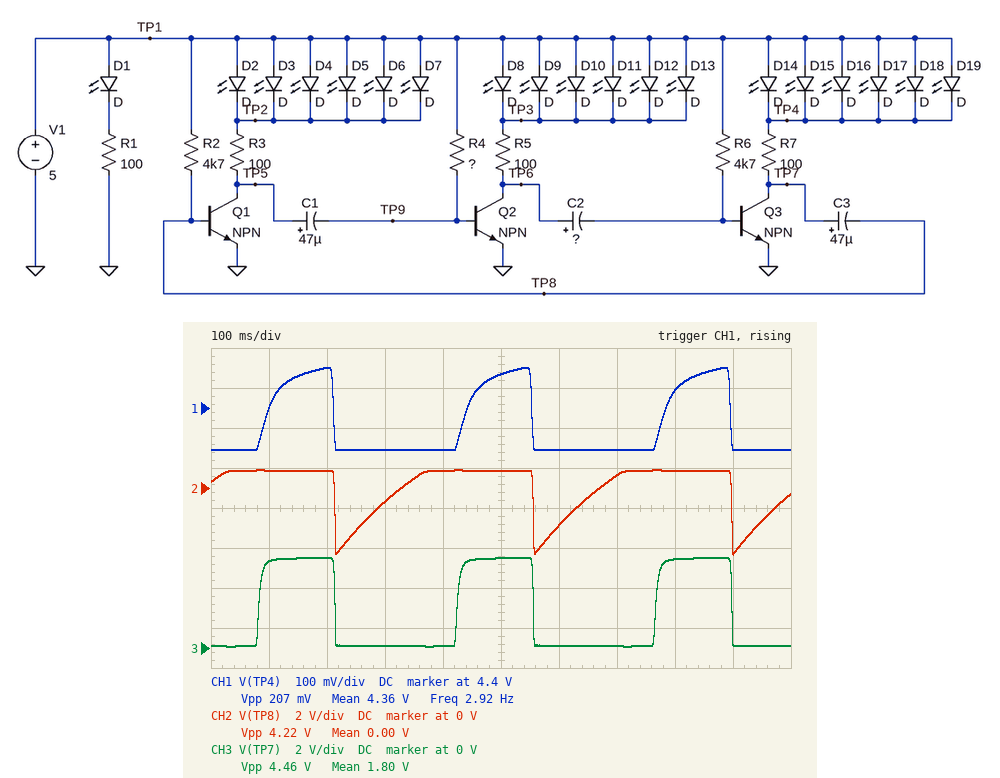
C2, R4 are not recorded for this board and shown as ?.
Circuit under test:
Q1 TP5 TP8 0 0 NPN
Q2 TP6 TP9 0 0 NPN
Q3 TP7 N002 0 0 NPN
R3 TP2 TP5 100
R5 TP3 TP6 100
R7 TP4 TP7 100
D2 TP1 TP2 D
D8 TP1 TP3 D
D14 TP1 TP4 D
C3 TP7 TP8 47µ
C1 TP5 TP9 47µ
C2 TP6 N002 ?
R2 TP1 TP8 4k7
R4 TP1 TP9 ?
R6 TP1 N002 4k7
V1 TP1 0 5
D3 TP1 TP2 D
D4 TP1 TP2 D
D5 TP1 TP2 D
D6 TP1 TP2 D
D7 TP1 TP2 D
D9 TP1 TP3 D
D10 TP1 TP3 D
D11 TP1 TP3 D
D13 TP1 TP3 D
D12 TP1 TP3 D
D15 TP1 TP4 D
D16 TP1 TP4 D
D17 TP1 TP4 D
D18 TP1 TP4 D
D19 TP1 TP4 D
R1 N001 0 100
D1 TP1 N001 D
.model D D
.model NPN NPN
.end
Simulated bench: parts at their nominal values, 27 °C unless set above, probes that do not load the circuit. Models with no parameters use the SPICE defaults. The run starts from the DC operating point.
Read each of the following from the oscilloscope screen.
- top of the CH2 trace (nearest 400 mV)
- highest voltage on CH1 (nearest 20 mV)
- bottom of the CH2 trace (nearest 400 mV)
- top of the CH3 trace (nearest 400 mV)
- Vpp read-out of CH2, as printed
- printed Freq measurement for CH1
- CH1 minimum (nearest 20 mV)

800 mV
4.50 V
-3.2 V
4.4 V
4.22 V
2.92 Hz
4.30 V
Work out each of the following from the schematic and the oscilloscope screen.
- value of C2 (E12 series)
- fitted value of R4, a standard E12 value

39 µF
1.5 kΩ
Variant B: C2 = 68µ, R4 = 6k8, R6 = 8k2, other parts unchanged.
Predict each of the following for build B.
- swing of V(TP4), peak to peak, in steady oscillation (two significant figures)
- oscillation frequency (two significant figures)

240 mV
1.3 Hz
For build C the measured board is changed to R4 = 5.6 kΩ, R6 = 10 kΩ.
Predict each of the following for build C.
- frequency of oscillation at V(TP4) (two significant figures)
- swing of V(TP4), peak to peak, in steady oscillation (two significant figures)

1.6 Hz
230 mV
